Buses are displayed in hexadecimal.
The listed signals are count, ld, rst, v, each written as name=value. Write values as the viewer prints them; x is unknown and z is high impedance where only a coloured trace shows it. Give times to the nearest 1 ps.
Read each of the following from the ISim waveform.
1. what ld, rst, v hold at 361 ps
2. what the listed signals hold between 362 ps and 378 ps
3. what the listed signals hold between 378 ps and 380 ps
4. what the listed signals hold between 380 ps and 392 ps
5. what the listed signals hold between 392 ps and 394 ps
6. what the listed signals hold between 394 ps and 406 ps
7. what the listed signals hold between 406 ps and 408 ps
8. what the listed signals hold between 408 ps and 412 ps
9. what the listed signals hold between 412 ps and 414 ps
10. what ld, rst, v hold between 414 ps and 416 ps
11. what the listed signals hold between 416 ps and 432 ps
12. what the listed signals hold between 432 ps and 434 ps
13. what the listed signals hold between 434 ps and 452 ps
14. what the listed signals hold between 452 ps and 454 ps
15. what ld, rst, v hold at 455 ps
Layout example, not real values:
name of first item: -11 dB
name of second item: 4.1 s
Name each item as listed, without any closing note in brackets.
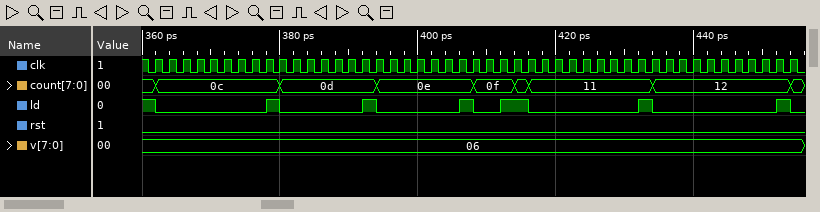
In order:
what ld, rst, v hold at 361 ps: ld=1, rst=0, v=06
what the listed signals hold between 362 ps and 378 ps: count=0c, ld=0, rst=0, v=06
what the listed signals hold between 378 ps and 380 ps: count=0c, ld=1, rst=0, v=06
what the listed signals hold between 380 ps and 392 ps: count=0d, ld=0, rst=0, v=06
what the listed signals hold between 392 ps and 394 ps: count=0d, ld=1, rst=0, v=06
what the listed signals hold between 394 ps and 406 ps: count=0e, ld=0, rst=0, v=06
what the listed signals hold between 406 ps and 408 ps: count=0e, ld=1, rst=0, v=06
what the listed signals hold between 408 ps and 412 ps: count=0f, ld=0, rst=0, v=06
what the listed signals hold between 412 ps and 414 ps: count=0f, ld=1, rst=0, v=06
what ld, rst, v hold between 414 ps and 416 ps: ld=1, rst=0, v=06
what the listed signals hold between 416 ps and 432 ps: count=11, ld=0, rst=0, v=06
what the listed signals hold between 432 ps and 434 ps: count=11, ld=1, rst=0, v=06
what the listed signals hold between 434 ps and 452 ps: count=12, ld=0, rst=0, v=06
what the listed signals hold between 452 ps and 454 ps: count=12, ld=1, rst=0, v=06
what ld, rst, v hold at 455 ps: ld=0, rst=0, v=06
